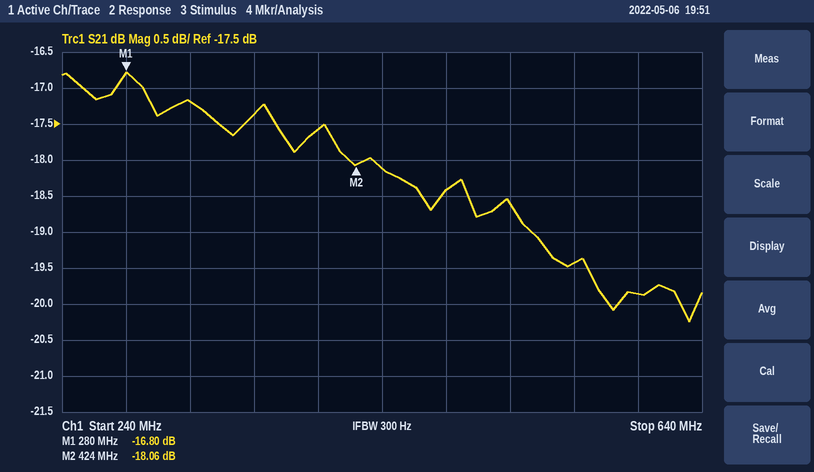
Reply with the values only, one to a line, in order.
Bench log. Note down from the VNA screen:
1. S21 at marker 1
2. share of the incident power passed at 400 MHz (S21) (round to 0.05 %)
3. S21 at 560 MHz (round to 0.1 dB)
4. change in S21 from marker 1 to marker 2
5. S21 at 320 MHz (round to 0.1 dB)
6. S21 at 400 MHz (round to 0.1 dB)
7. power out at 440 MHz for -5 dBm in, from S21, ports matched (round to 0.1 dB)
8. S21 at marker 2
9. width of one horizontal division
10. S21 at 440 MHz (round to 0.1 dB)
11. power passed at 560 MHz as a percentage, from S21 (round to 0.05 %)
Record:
-16.80 dB
1.75 %
-19.4 dB
-1.26 dB
-17.2 dB
-17.6 dB
-23.1 dBm
-18.06 dB
40 MHz
-18.1 dB
1.15 %
